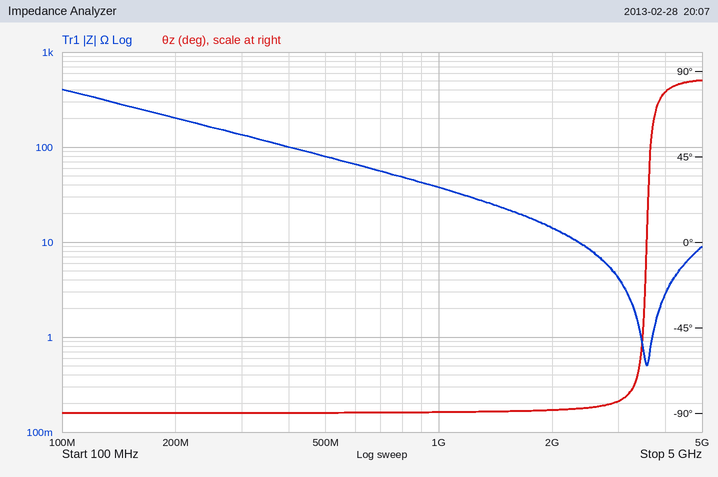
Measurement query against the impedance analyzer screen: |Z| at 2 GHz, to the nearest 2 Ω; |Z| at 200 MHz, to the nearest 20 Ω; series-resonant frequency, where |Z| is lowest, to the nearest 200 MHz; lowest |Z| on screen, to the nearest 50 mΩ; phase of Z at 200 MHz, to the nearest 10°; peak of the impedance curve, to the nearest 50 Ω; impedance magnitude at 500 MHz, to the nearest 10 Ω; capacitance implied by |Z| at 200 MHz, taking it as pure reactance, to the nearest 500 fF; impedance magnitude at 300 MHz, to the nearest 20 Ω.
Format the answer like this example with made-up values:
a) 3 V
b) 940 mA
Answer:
a) 14 Ω
b) 200 Ω
c) 3.6 GHz
d) 500 mΩ
e) -90°
f) 400 Ω
g) 80 Ω
h) 4.0 pF
i) 140 Ω
